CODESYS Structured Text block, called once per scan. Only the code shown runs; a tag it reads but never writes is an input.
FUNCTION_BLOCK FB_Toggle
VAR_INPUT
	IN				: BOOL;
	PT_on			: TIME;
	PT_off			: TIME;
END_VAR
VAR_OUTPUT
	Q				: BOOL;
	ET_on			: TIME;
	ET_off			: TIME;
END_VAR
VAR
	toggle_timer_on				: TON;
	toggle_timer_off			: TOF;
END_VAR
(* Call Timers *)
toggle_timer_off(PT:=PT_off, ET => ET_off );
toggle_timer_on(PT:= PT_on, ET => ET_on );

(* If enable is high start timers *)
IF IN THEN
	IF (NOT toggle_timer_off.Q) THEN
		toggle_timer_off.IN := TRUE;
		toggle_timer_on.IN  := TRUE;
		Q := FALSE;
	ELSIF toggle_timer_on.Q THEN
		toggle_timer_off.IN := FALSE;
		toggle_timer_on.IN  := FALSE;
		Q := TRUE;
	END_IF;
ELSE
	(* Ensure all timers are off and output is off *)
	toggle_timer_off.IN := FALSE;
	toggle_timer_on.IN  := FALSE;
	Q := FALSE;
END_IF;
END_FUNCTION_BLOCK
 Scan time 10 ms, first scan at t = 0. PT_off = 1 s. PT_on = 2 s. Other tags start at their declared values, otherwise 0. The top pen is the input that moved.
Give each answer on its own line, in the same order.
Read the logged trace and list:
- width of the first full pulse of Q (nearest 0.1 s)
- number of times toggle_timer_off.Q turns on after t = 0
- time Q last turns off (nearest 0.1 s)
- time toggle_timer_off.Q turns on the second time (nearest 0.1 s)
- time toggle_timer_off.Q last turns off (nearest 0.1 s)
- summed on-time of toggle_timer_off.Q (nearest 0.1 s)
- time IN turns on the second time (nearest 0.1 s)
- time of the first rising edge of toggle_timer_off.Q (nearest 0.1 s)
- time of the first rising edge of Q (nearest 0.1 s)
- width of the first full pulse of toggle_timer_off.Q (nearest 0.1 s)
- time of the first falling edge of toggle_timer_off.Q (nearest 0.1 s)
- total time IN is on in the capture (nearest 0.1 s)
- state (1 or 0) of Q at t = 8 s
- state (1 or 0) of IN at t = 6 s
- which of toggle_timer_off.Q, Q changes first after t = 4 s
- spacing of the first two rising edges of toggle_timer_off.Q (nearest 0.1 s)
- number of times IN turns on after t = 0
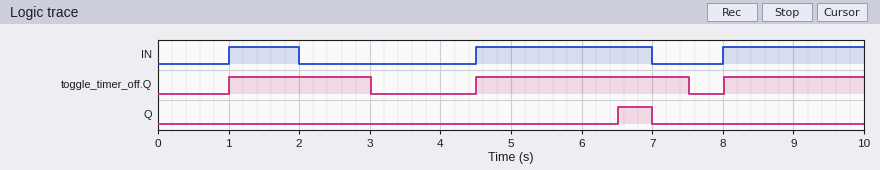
0.5 s
3
7.0 s
4.5 s
7.5 s
7.0 s
4.5 s
1.0 s
6.5 s
2.0 s
3.0 s
5.5 s
0
1
toggle_timer_off.Q
3.5 s
3
